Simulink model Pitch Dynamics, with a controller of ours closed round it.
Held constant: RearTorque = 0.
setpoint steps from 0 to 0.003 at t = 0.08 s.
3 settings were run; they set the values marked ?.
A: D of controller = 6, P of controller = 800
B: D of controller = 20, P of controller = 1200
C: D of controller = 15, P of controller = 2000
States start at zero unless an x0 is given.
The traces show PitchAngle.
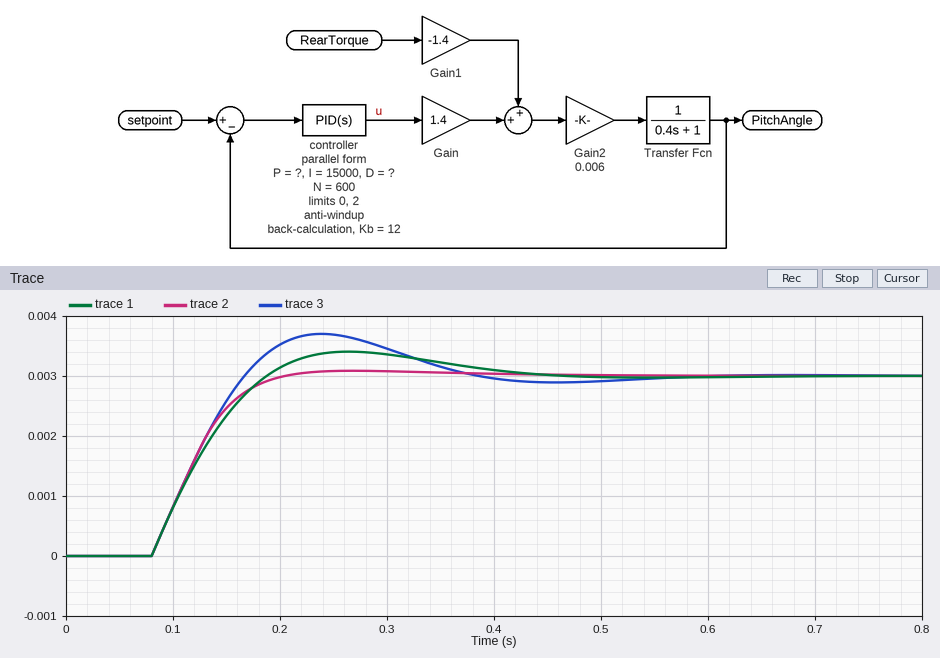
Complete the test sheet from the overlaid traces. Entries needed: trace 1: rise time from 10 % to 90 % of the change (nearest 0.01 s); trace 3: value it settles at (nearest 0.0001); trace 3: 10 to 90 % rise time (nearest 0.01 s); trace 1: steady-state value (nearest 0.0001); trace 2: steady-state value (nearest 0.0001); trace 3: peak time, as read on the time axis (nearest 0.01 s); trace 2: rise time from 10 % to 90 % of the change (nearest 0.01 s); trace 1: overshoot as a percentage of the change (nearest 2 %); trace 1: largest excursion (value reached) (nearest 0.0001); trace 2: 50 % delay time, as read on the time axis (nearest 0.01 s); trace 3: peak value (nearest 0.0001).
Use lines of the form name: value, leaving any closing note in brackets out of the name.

trace 1: rise time from 10 % to 90 % of the change: 0.08 s
trace 3: value it settles at: 0.0030
trace 3: 10 to 90 % rise time: 0.07 s
trace 1: steady-state value: 0.0030
trace 2: steady-state value: 0.0030
trace 3: peak time, as read on the time axis: 0.24 s
trace 2: rise time from 10 % to 90 % of the change: 0.08 s
trace 1: overshoot as a percentage of the change: 14 %
trace 1: largest excursion (value reached): 0.0034
trace 2: 50 % delay time, as read on the time axis: 0.12 s
trace 3: peak value: 0.0037
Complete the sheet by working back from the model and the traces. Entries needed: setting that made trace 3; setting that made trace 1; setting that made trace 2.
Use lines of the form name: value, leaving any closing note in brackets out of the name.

setting that made trace 3: A
setting that made trace 1: B
setting that made trace 2: C
